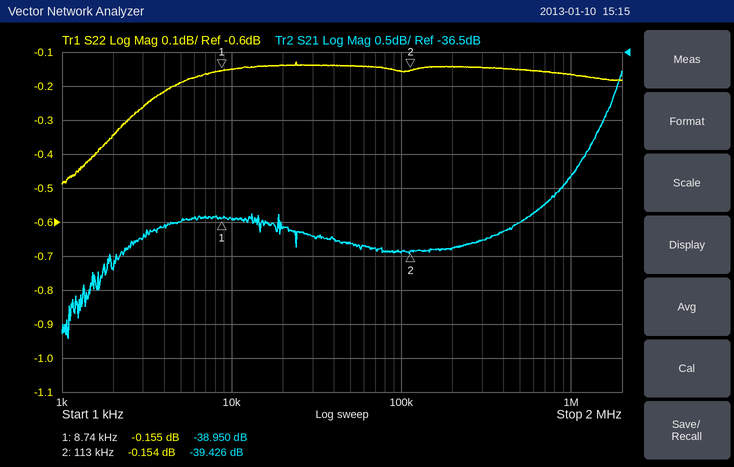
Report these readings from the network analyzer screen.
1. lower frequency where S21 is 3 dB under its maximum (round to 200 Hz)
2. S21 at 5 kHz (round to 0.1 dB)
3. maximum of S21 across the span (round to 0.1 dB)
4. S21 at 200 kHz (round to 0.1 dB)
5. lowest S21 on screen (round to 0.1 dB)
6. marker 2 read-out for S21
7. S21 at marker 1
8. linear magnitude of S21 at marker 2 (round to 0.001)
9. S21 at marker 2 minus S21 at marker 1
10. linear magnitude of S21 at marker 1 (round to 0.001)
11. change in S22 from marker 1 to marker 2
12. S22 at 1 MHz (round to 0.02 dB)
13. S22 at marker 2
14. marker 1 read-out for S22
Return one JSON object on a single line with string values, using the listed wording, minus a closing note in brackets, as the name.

{"lower frequency where S21 is 3 dB under its maximum": "1.8 kHz", "S21 at 5 kHz": "-39.0 dB", "maximum of S21 across the span": "-36.8 dB", "S21 at 200 kHz": "-39.4 dB", "lowest S21 on screen": "-40.7 dB", "marker 2 read-out for S21": "-39.426 dB", "S21 at marker 1": "-38.950 dB", "linear magnitude of S21 at marker 2": "0.011", "S21 at marker 2 minus S21 at marker 1": "-0.476 dB", "linear magnitude of S21 at marker 1": "0.011", "change in S22 from marker 1 to marker 2": "0.001 dB", "S22 at 1 MHz": "-0.16 dB", "S22 at marker 2": "-0.154 dB", "marker 1 read-out for S22": "-0.155 dB"}
